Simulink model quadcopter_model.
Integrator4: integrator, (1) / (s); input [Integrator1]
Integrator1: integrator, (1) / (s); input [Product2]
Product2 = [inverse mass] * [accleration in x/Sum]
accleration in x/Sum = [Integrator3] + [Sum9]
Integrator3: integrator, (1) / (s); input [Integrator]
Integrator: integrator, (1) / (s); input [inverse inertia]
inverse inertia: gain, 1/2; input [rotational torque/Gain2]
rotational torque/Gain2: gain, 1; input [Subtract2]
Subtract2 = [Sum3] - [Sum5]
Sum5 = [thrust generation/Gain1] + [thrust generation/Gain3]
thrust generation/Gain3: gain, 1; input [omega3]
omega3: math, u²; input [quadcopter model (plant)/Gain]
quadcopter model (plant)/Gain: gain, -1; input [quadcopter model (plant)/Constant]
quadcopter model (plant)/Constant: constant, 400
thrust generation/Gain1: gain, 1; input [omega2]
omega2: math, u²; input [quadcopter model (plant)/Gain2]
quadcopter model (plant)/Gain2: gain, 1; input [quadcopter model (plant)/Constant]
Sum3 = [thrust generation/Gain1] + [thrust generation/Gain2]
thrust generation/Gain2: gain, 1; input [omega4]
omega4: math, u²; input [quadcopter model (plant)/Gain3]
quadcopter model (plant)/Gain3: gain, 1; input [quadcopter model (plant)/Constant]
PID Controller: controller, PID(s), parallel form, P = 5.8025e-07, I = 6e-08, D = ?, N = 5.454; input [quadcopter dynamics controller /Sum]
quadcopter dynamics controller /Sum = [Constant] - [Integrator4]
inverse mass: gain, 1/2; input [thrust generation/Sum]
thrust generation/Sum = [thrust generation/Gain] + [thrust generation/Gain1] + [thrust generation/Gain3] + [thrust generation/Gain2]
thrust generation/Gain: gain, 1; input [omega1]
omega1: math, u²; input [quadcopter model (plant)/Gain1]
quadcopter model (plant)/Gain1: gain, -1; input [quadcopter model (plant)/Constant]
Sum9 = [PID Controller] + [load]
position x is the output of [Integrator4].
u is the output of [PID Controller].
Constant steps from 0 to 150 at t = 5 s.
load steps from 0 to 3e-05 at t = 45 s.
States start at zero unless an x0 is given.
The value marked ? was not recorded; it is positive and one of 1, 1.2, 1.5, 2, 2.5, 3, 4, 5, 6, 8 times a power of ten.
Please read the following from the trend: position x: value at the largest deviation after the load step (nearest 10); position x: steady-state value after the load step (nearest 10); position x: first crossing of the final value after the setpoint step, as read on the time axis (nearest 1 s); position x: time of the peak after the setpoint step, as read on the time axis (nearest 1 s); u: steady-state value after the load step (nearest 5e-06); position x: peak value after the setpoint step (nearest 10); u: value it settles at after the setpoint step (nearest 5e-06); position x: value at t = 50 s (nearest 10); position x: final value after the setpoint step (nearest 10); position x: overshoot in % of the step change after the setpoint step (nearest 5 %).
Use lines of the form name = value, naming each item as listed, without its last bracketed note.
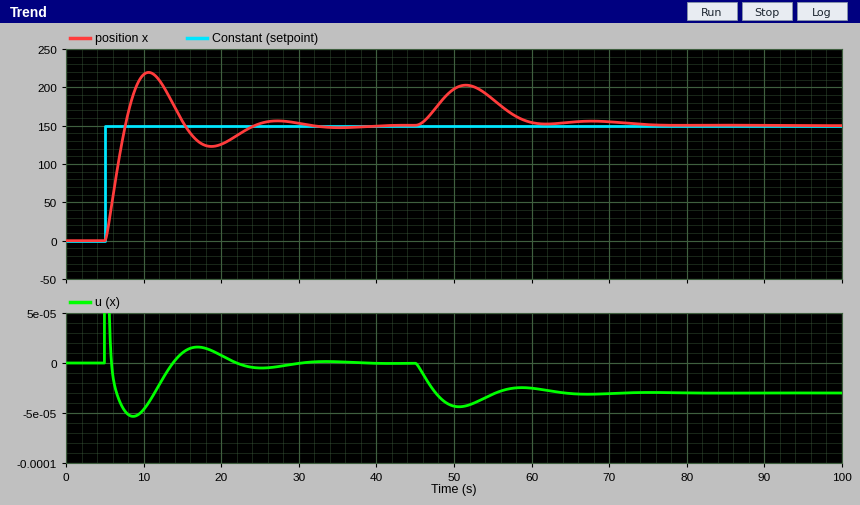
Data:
position x: value at the largest deviation after the load step = 200
position x: steady-state value after the load step = 150
position x: first crossing of the final value after the setpoint step, as read on the time axis = 8 s
position x: time of the peak after the setpoint step, as read on the time axis = 11 s
u: steady-state value after the load step = -0.000030
position x: peak value after the setpoint step = 220
u: value it settles at after the setpoint step = 0.000000
position x: value at t = 50 s = 200
position x: final value after the setpoint step = 150
position x: overshoot in % of the step change after the setpoint step = 45 %
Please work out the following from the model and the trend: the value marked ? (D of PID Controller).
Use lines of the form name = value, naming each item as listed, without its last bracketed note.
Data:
the value marked ? = 1.2e-06
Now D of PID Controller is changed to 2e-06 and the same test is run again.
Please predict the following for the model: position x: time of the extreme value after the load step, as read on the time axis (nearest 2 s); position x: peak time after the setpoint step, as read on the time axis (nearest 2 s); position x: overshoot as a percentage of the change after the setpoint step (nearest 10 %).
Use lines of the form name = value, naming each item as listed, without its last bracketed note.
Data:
position x: time of the extreme value after the load step, as read on the time axis = 52 s
position x: peak time after the setpoint step, as read on the time axis = 10 s
position x: overshoot as a percentage of the change after the setpoint step = 30 %
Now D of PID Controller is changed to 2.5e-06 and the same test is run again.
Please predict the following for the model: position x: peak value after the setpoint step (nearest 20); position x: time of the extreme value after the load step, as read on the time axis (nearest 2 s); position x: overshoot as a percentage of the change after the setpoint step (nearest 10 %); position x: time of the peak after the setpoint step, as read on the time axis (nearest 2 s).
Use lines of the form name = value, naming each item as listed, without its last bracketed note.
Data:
position x: peak value after the setpoint step = 180
position x: time of the extreme value after the load step, as read on the time axis = 52 s
position x: overshoot as a percentage of the change after the setpoint step = 20 %
position x: time of the peak after the setpoint step, as read on the time axis = 10 s
